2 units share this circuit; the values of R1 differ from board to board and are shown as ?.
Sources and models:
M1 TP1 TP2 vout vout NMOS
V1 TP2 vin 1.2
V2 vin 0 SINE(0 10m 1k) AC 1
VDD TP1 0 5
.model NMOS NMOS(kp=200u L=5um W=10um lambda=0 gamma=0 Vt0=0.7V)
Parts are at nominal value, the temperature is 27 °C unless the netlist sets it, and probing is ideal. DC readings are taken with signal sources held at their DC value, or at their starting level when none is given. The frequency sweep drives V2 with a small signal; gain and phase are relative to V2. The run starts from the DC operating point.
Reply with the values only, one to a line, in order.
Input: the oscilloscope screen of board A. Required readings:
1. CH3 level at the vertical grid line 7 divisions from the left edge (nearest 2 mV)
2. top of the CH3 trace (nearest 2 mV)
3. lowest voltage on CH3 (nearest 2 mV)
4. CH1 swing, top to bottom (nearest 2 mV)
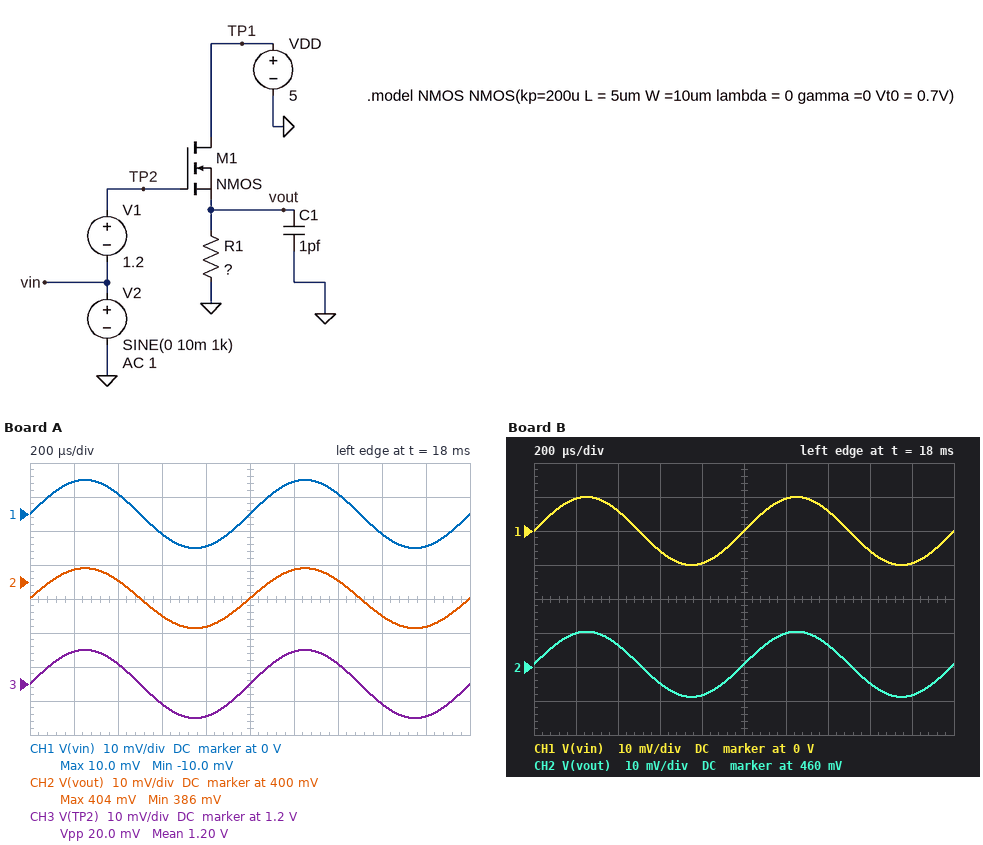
1.206 V
1.210 V
1.190 V
20 mV
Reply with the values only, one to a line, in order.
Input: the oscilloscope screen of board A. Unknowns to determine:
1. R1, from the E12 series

180 kΩ
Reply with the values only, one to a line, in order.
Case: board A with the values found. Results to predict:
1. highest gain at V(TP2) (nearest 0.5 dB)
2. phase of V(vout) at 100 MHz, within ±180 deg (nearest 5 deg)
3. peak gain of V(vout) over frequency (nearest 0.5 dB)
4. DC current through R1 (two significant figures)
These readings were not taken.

0 dB
-85 deg
-1.0 dB
2.2 µA
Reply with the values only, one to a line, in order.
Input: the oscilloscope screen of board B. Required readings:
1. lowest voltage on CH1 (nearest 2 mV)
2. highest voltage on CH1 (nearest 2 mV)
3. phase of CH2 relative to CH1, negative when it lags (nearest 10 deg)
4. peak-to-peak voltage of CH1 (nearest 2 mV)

-10 mV
10 mV
0 deg
20 mV
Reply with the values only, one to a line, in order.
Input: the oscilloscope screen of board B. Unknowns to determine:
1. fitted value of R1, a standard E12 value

1.5 MΩ
